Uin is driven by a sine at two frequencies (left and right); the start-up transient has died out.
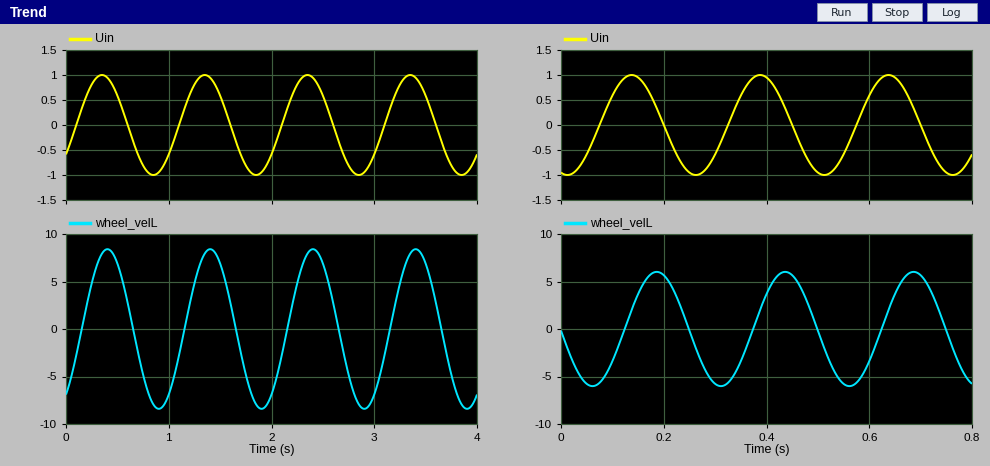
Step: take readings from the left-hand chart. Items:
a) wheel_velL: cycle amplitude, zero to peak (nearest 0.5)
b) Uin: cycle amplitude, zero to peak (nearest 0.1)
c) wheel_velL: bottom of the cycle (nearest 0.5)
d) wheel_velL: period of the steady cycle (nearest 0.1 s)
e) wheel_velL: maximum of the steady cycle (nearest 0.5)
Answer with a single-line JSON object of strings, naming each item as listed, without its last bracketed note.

{"wheel_velL: cycle amplitude, zero to peak": "8.5", "Uin: cycle amplitude, zero to peak": "1.0", "wheel_velL: bottom of the cycle": "-8.5", "wheel_velL: period of the steady cycle": "1.0 s", "wheel_velL: maximum of the steady cycle": "8.5"}
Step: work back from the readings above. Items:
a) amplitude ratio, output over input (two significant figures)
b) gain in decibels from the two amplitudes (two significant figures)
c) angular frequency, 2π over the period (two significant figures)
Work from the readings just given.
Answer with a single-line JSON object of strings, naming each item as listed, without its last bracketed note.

{"amplitude ratio, output over input": "8.5", "gain in decibels from the two amplitudes": "19 dB", "angular frequency, 2π over the period": "6.3 rad/s"}
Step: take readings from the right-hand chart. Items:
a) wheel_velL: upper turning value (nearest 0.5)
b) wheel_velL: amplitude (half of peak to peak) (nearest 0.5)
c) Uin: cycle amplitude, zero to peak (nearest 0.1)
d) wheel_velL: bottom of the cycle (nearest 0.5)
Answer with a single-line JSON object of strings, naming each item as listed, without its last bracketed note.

{"wheel_velL: upper turning value": "6.0", "wheel_velL: amplitude (half of peak to peak)": "6.0", "Uin: cycle amplitude, zero to peak": "1.0", "wheel_velL: bottom of the cycle": "-6.0"}
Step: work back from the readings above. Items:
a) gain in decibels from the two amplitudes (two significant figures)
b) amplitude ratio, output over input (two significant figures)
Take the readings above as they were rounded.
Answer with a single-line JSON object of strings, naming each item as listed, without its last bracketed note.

{"gain in decibels from the two amplitudes": "16 dB", "amplitude ratio, output over input": "6.0"}
